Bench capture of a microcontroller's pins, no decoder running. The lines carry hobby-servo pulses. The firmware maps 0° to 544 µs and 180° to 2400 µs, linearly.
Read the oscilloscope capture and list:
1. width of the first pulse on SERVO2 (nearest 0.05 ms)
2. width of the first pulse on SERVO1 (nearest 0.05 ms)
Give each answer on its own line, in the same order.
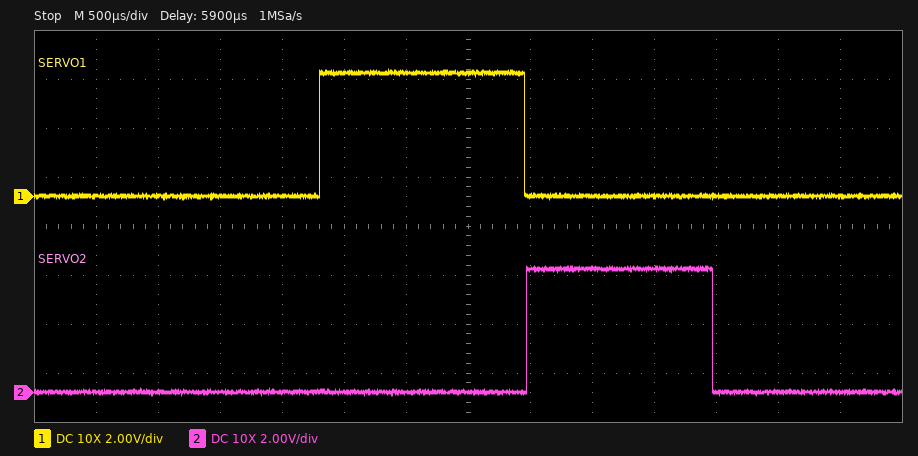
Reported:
1.50 ms
1.65 ms
